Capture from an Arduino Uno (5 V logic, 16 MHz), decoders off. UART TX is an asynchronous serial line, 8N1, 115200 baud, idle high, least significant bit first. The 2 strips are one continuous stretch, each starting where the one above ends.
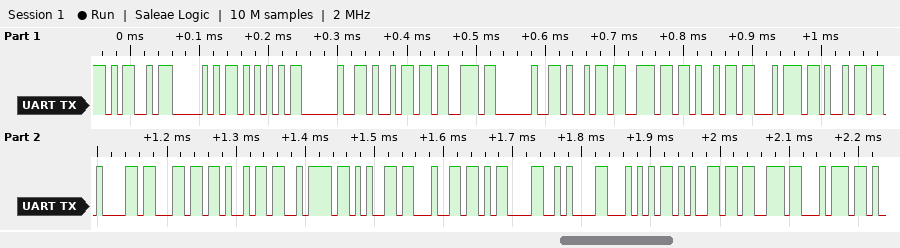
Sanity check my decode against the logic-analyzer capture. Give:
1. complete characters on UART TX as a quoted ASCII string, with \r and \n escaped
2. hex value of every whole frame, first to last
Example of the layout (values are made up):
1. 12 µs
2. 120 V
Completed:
1. "MPU is initialized\r\nTest"
2. 0x4D 0x50 0x55 0x20 0x69 0x73 0x20 0x69 0x6E 0x69 0x74 0x69 0x61 0x6C 0x69 0x7A 0x65 0x64 0x0D 0x0A 0x54 0x65 0x73 0x74
